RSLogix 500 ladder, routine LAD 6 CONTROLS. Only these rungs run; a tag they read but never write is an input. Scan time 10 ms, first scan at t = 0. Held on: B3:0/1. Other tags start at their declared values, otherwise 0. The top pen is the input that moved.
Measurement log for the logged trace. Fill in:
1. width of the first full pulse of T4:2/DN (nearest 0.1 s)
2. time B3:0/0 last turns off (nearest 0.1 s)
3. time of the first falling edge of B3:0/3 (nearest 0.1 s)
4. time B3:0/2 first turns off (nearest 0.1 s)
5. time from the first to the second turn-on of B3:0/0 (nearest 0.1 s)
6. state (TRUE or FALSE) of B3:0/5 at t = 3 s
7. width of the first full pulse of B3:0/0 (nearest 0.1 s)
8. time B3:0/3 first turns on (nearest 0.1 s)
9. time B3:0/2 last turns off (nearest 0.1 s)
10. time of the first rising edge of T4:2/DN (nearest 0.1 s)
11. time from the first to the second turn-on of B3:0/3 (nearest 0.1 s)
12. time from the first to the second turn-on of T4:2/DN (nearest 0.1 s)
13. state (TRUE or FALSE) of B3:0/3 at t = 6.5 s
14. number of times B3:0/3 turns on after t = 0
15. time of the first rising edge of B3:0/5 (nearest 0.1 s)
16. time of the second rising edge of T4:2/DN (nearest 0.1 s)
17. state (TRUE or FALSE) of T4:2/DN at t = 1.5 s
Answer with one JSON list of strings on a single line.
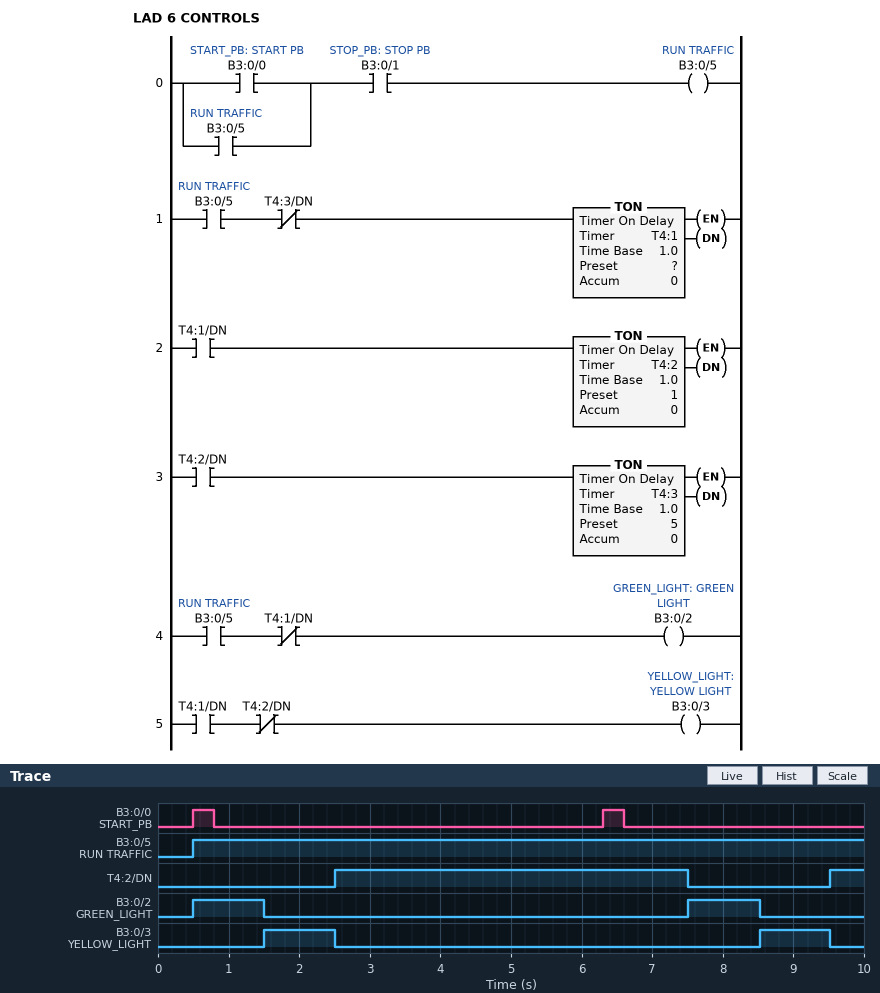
["5.0 s", "6.6 s", "2.5 s", "1.5 s", "5.8 s", "TRUE", "0.3 s", "1.5 s", "8.5 s", "2.5 s", "7.0 s", "7.0 s", "FALSE", "2", "0.5 s", "9.5 s", "FALSE"]
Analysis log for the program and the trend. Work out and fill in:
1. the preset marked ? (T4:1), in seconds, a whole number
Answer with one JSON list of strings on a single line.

["1 s"]
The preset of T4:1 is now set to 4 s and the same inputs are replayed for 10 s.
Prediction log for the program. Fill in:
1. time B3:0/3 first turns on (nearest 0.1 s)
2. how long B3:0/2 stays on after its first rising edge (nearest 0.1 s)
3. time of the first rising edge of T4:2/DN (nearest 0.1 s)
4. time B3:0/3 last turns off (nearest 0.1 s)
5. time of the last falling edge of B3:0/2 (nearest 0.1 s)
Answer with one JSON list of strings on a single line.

["4.5 s", "4.0 s", "5.5 s", "5.5 s", "4.5 s"]
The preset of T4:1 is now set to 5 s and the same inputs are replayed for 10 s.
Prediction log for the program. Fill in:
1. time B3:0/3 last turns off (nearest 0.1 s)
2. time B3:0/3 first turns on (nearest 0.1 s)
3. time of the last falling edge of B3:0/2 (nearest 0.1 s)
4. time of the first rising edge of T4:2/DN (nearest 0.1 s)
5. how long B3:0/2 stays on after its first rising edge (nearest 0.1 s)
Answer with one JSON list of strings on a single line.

["6.5 s", "5.5 s", "5.5 s", "6.5 s", "5.0 s"]
